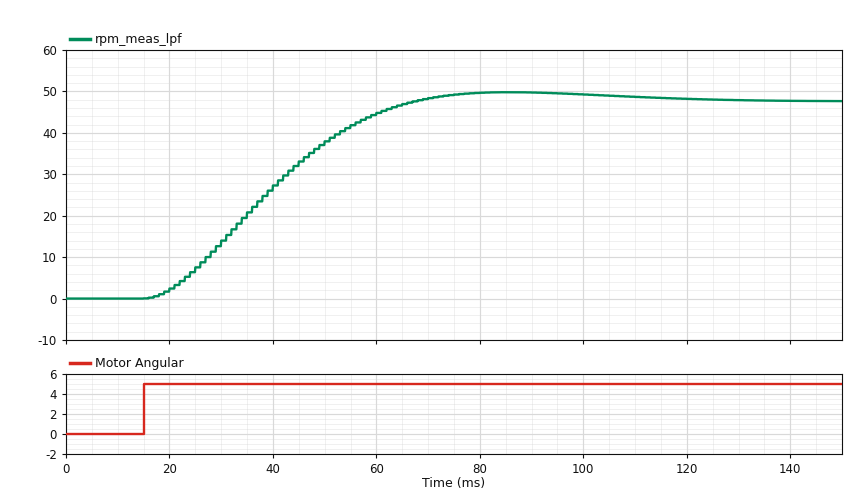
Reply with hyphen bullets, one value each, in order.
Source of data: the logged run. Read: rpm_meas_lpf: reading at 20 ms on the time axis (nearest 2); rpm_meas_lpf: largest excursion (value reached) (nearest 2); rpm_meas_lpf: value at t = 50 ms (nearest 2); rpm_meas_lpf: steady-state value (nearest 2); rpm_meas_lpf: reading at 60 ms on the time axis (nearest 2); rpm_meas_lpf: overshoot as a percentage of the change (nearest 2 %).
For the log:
- 2
- 50
- 38
- 48
- 44
- 4 %
